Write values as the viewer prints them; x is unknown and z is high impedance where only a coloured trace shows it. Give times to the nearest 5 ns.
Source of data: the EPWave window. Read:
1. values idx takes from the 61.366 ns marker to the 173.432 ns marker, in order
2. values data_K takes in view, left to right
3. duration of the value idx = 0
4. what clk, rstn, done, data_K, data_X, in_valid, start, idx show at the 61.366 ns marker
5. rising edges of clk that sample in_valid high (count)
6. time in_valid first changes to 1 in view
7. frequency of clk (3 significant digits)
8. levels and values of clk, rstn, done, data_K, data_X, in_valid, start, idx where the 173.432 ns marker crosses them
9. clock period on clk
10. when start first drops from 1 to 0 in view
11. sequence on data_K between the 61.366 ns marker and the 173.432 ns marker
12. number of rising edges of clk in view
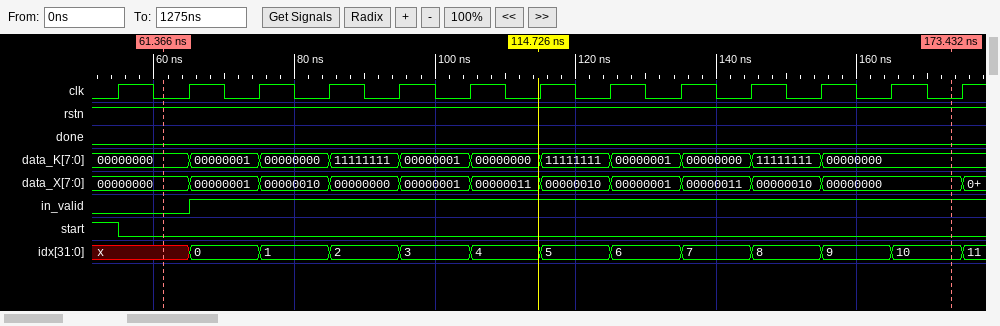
x, 0, 1, 2, 3, 4, 5, 6, 7, 8, 9, 10
00000000, 00000001, 00000000, 11111111, 00000001, 00000000, 11111111, 00000001, 00000000, 11111111, 00000000
10 ns
clk=0, rstn=1, done=0, data_K=00000000, data_X=00000000, in_valid=0, start=0, idx=x
11
65 ns
100 MHz
clk=0, rstn=1, done=0, data_K=00000000, data_X=00000000, in_valid=1, start=0, idx=10
10 ns
55 ns
00000000, 00000001, 00000000, 11111111, 00000001, 00000000, 11111111, 00000001, 00000000, 11111111, 00000000
13
